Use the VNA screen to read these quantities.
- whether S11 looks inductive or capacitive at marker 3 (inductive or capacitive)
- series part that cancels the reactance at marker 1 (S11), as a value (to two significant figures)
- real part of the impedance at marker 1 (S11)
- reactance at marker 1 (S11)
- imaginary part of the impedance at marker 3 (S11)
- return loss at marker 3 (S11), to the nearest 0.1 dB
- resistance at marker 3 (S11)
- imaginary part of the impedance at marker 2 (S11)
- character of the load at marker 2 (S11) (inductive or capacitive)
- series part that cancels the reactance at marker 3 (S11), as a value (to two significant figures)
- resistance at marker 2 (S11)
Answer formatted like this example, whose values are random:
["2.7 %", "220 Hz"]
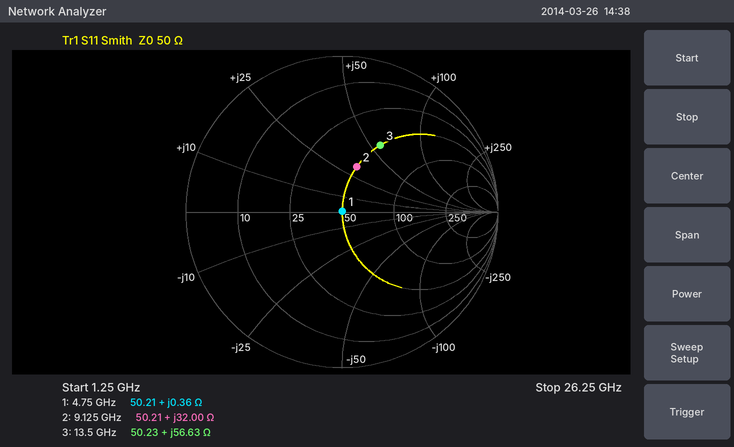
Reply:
["inductive", "93 pF", "50.21 Ω", "+0.36 Ω", "+56.63 Ω", "6.2 dB", "50.23 Ω", "+32.00 Ω", "inductive", "210 fF", "50.21 Ω"]
